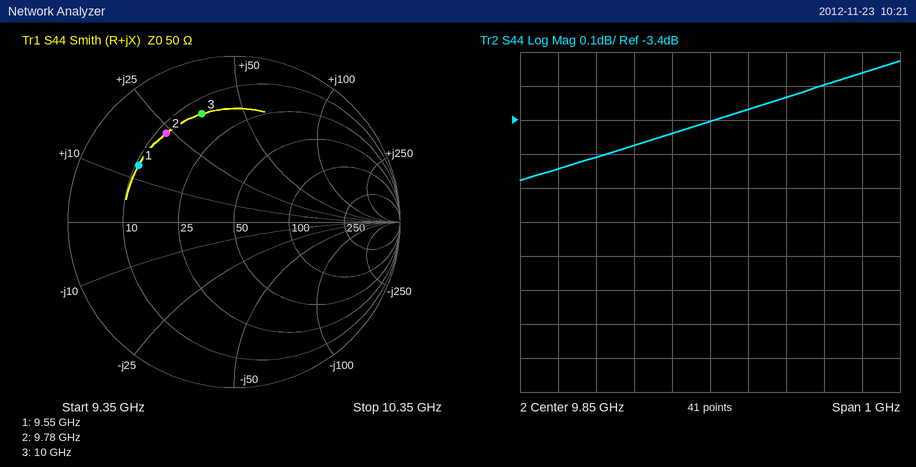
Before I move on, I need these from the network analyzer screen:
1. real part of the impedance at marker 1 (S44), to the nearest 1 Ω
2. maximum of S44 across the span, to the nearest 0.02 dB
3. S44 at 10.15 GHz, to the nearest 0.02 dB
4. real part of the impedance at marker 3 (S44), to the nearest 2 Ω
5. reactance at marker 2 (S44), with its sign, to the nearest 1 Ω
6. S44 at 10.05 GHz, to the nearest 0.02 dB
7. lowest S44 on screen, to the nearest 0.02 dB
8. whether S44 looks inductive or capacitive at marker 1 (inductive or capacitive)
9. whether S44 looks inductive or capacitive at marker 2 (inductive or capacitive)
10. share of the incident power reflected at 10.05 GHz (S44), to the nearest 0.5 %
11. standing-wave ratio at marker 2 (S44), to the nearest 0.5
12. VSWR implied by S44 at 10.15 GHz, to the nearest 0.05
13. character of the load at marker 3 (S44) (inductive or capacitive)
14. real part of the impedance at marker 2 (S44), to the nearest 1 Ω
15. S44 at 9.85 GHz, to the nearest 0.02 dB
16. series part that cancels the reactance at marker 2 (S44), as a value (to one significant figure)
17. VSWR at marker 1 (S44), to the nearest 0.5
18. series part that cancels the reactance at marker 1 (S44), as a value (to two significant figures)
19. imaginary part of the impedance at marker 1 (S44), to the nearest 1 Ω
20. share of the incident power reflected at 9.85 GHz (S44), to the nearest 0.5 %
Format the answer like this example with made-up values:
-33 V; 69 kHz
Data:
11 Ω; -3.22 dB; -3.30 dB; 14 Ω; +24 Ω; -3.34 dB; -3.58 dB; inductive; inductive; 46.5 %; 5.0; 5.35; inductive; 12 Ω; -3.40 dB; 700 fF; 5.0; 1.3 pF; +13 Ω; 45.5 %
